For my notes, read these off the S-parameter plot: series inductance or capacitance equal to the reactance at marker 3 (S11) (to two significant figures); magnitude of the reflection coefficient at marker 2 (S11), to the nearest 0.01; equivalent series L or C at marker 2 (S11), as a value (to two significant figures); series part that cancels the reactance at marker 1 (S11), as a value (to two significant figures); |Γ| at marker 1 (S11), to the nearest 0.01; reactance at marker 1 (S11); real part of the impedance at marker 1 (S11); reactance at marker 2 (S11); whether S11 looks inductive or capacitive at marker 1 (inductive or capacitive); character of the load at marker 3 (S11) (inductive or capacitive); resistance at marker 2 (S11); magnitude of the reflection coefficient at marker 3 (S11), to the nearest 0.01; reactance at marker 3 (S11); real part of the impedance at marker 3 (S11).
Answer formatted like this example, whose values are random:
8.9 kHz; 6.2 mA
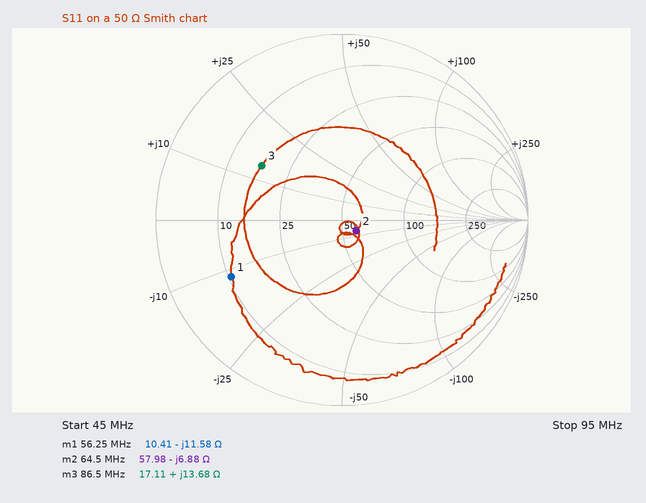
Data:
25 nH; 0.10; 360 pF; 33 nH; 0.67; -11.58 Ω; 10.41 Ω; -6.88 Ω; capacitive; inductive; 57.98 Ω; 0.52; +13.68 Ω; 17.11 Ω
